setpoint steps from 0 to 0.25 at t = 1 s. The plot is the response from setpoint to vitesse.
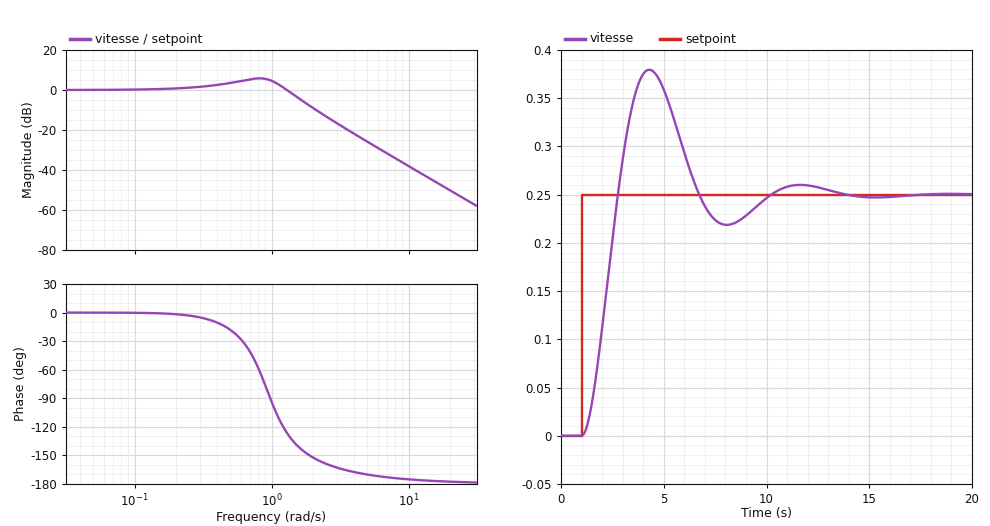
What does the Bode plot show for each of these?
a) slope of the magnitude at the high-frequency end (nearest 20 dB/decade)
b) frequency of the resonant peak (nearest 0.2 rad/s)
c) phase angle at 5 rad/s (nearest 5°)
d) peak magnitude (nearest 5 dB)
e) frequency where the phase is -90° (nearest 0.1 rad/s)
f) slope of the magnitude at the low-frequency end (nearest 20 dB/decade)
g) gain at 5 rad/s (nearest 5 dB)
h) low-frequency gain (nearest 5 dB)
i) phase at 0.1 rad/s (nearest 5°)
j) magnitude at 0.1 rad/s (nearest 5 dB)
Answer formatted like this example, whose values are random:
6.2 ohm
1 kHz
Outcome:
-40 dB/decade
0.8 rad/s
-170°
5 dB
1.0 rad/s
0 dB/decade
-25 dB
0 dB
0°
0 dB
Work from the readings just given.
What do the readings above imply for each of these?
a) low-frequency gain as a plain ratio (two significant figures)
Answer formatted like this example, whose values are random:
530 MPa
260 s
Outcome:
1.0
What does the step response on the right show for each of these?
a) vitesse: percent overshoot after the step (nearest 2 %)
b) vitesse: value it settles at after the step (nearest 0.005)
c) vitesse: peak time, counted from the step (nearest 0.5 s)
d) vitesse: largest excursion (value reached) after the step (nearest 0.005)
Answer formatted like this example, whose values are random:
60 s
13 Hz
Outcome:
52 %
0.250
3.5 s
0.380
